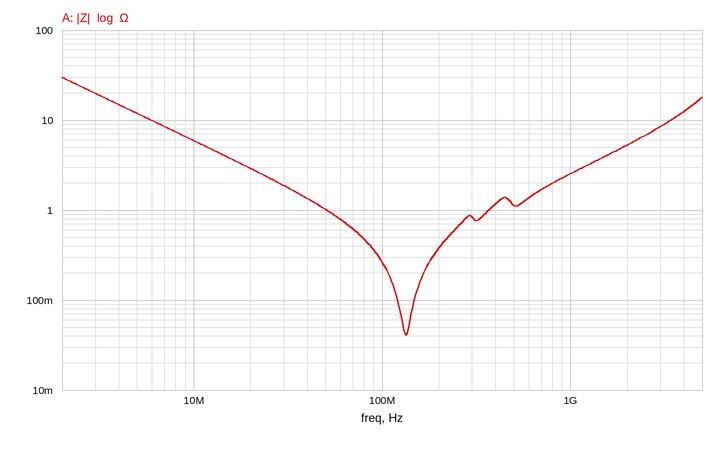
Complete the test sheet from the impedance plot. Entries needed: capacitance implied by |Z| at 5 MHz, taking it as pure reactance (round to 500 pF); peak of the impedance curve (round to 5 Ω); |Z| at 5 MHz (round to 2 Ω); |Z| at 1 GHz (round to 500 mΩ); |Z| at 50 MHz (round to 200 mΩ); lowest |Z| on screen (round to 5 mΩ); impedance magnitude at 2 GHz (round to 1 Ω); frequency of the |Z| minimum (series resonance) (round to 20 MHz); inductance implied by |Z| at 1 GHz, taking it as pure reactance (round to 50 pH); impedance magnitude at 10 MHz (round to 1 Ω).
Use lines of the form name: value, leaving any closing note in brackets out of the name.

capacitance implied by |Z| at 5 MHz, taking it as pure reactance: 2.5 nF
peak of the impedance curve: 30 Ω
|Z| at 5 MHz: 12 Ω
|Z| at 1 GHz: 2.5 Ω
|Z| at 50 MHz: 1.0 Ω
lowest |Z| on screen: 40 mΩ
impedance magnitude at 2 GHz: 5 Ω
frequency of the |Z| minimum (series resonance): 140 MHz
inductance implied by |Z| at 1 GHz, taking it as pure reactance: 400 pH
impedance magnitude at 10 MHz: 6 Ω
